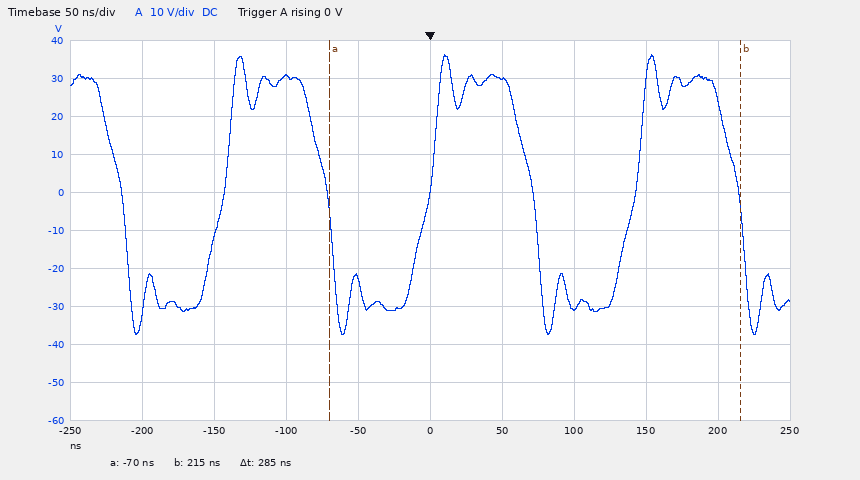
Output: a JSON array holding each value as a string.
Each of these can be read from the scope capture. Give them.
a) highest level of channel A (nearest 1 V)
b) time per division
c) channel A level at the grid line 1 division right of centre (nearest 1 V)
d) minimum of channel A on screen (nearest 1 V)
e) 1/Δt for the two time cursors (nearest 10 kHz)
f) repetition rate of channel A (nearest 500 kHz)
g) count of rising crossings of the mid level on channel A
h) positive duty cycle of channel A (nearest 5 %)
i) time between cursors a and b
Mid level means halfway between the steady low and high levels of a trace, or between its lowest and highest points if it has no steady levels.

["36 V", "50 ns", "30 V", "-37 V", "3.51 MHz", "7.0 MHz", "3", "50 %", "285 ns"]
